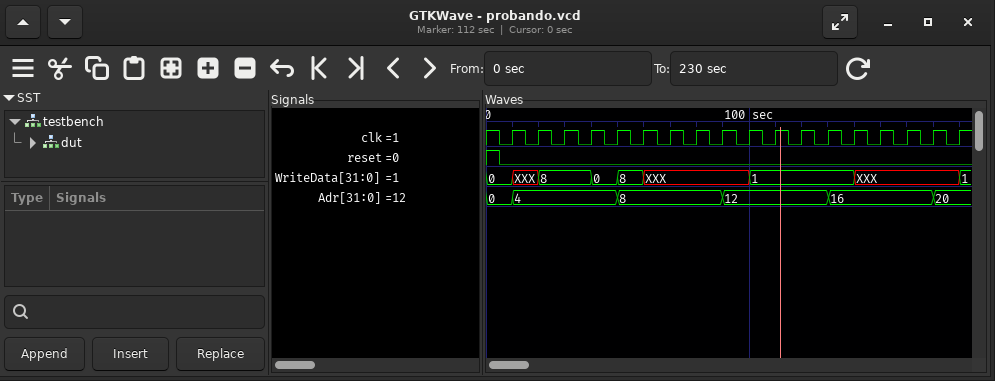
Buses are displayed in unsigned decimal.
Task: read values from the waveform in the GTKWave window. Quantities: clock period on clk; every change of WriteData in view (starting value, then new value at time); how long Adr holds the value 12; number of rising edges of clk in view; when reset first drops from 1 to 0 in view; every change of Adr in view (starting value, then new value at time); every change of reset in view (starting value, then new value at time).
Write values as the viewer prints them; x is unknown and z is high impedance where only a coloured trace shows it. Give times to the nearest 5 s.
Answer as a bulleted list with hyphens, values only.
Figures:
- 10 s
- 0, XXX at 10 s, 8 at 20 s, 0 at 40 s, 8 at 50 s, XXX at 60 s, 1 at 100 s, XXX at 140 s, 1 at 180 s
- 40 s
- 18
- 5 s
- 0, 4 at 10 s, 8 at 50 s, 12 at 90 s, 16 at 130 s, 20 at 170 s
- 1, 0 at 5 s
